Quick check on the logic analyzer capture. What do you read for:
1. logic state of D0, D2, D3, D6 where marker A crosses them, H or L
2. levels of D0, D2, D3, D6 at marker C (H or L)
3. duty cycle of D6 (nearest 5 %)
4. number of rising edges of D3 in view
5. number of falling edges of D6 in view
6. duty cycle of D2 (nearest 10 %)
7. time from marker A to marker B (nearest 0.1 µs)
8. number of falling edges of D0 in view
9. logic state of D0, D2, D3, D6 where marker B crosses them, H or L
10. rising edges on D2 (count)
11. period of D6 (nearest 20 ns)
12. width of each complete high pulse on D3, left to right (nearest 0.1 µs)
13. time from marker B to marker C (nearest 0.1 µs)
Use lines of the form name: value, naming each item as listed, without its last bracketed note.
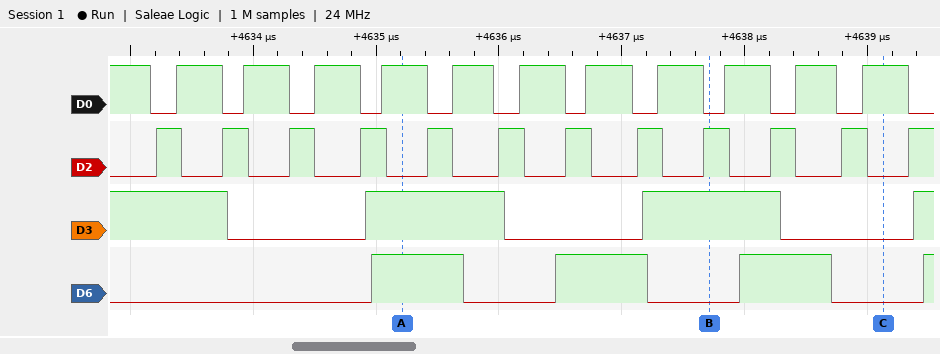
logic state of D0, D2, D3, D6 where marker A crosses them, H or L: D0=H, D2=L, D3=H, D6=H
levels of D0, D2, D3, D6 at marker C: D0=H, D2=L, D3=L, D6=L
duty cycle of D6: 50 %
number of rising edges of D3 in view: 3
number of falling edges of D6 in view: 3
duty cycle of D2: 40 %
time from marker A to marker B: 2.5 µs
number of falling edges of D0 in view: 12
logic state of D0, D2, D3, D6 where marker B crosses them, H or L: D0=L, D2=H, D3=H, D6=L
rising edges on D2: 12
period of D6: 1500 ns
width of each complete high pulse on D3, left to right: 1.1 µs, 1.1 µs
time from marker B to marker C: 1.4 µs
